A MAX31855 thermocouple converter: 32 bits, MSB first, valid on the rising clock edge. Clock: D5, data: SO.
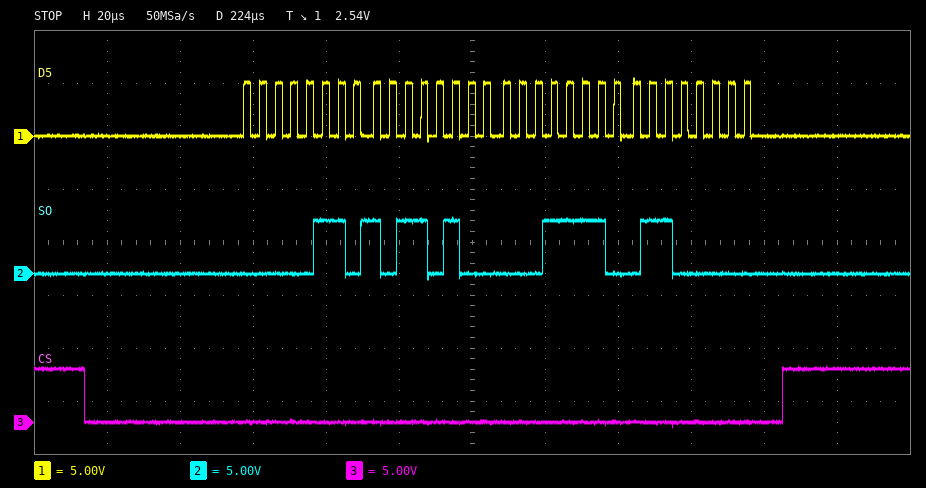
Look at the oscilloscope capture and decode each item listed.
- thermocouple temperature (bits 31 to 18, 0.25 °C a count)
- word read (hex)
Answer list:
107.25 °C
0x06B41E60
